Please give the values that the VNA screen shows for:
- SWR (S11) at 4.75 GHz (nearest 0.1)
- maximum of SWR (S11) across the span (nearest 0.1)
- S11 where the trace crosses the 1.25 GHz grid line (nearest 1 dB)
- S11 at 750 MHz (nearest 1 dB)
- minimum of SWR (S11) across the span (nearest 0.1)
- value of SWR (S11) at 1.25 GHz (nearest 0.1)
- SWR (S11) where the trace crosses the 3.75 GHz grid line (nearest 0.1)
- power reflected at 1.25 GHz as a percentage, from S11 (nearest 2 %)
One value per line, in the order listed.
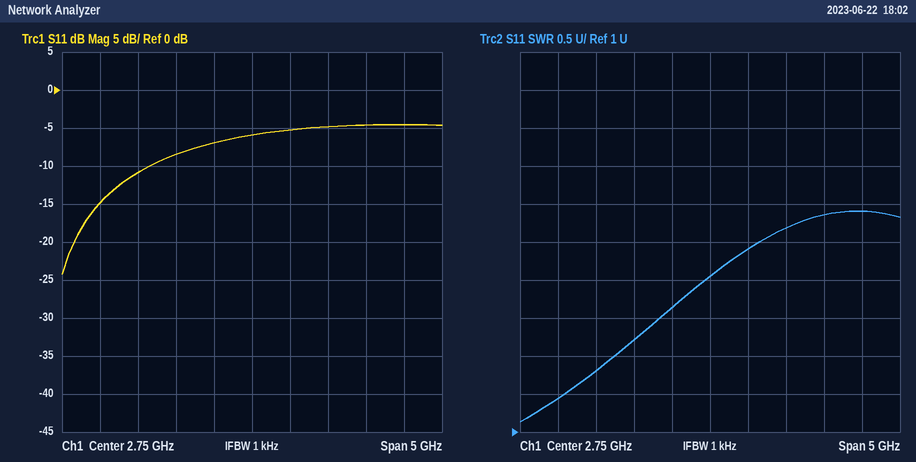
3.9
3.9
-11 dB
-15 dB
1.1
1.8
3.7
8 %
